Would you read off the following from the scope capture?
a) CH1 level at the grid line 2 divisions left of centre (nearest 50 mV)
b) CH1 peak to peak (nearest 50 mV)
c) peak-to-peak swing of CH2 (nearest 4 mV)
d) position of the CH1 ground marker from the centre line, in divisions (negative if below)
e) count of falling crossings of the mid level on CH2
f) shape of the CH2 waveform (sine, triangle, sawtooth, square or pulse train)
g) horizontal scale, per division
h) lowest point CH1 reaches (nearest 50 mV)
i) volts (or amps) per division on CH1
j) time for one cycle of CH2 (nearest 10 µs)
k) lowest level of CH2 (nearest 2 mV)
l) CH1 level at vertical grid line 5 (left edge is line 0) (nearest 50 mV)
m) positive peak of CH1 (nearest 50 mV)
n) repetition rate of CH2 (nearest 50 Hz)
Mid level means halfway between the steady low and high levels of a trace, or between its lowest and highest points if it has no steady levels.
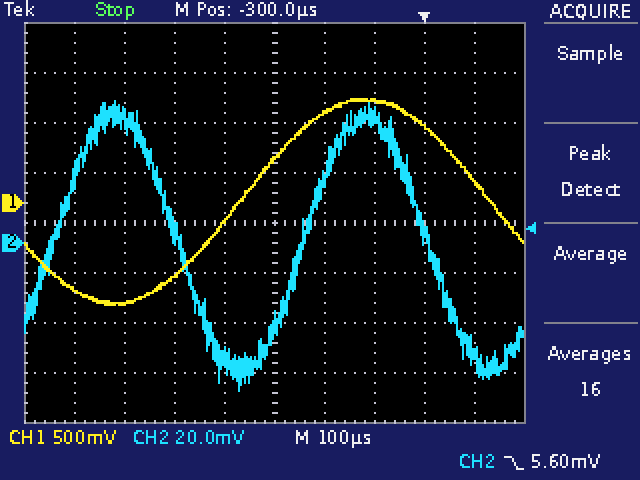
-750 mV
2.05 V
116 mV
+0.4 div
2
sine
100 µs
-1.00 V
500 mV
500 µs
-60 mV
450 mV
1.05 V
2.00 kHz
